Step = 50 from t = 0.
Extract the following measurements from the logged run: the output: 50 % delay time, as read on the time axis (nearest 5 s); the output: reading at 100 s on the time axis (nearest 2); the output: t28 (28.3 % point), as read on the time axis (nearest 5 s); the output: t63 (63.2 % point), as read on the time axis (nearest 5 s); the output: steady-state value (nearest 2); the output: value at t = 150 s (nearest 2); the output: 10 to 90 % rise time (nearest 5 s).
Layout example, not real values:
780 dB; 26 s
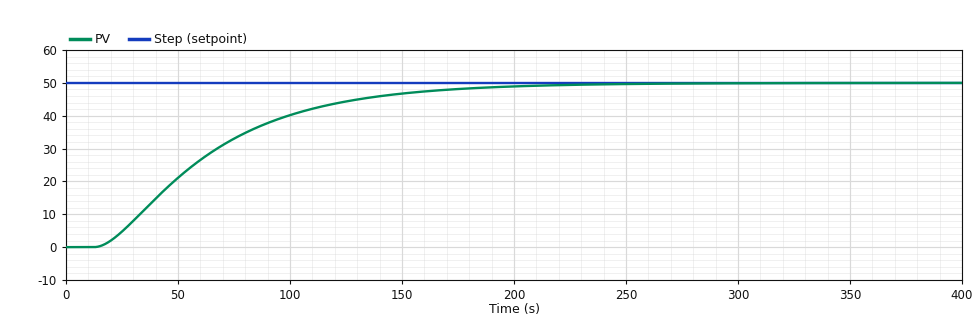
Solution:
55 s; 40; 40 s; 70 s; 50; 46; 105 s
